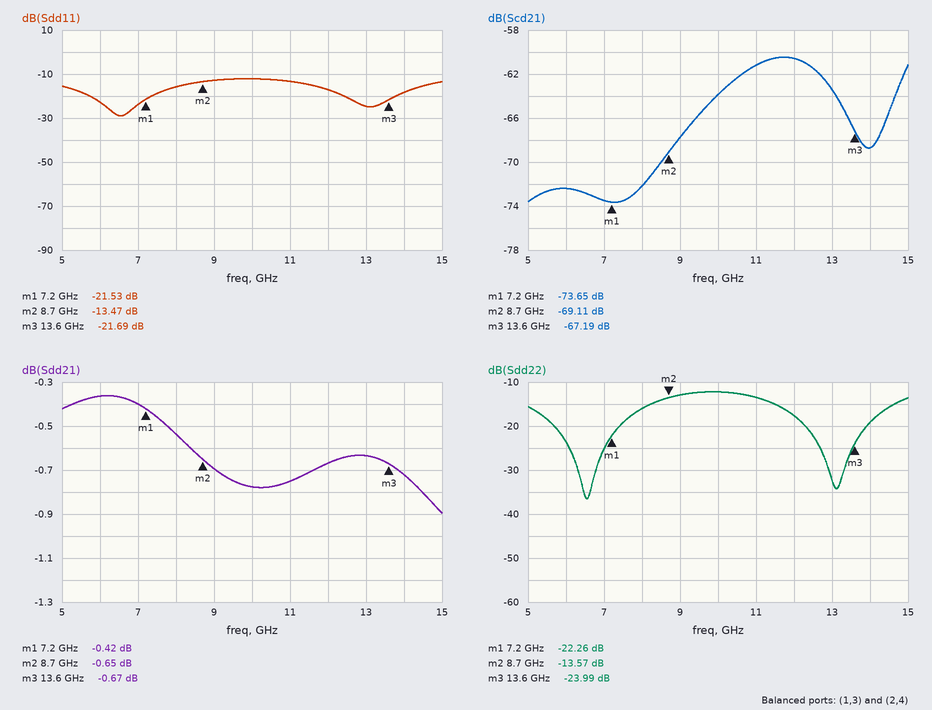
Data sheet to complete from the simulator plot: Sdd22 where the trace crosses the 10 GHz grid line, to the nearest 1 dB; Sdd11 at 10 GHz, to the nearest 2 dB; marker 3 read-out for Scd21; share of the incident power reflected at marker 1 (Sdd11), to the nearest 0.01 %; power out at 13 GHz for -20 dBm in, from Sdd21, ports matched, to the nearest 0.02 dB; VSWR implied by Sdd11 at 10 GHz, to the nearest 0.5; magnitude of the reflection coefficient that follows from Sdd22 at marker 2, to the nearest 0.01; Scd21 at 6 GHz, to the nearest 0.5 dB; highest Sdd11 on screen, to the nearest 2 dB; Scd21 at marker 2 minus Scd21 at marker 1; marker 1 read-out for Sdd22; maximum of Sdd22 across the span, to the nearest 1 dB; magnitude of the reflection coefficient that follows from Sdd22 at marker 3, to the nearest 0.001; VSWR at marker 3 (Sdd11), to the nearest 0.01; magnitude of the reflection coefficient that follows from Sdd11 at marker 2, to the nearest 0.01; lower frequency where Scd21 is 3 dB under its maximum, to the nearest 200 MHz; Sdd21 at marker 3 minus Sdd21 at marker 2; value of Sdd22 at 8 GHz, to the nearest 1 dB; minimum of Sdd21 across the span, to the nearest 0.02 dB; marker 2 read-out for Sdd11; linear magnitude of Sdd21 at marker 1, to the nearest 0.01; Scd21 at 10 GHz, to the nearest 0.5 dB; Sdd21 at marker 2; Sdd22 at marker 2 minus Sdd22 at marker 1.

-12 dB
-12 dB
-67.19 dB
0.70 %
-20.64 dBm
1.5
0.21
-72.5 dB
-12 dB
4.54 dB
-22.26 dB
-12 dB
0.063
1.18
0.21
10.2 GHz
-0.02 dB
-16 dB
-0.90 dB
-13.47 dB
0.95
-64.0 dB
-0.65 dB
8.69 dB
